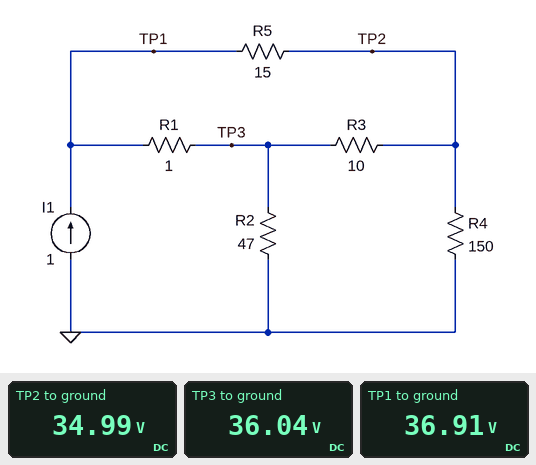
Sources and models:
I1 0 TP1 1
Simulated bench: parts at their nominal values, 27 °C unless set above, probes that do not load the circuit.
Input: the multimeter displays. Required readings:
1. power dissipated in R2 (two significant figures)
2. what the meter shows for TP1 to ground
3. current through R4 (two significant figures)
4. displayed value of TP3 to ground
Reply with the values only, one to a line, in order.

28 W
36.91 V
230 mA
36.04 V
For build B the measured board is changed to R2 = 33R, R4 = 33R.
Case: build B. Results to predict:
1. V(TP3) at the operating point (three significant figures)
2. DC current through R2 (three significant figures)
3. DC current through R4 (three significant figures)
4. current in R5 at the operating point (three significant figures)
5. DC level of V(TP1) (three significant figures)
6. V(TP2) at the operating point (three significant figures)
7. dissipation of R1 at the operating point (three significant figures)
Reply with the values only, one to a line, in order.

17.7 V
537 mA
463 mA
216 mA
18.5 V
15.3 V
614 mW
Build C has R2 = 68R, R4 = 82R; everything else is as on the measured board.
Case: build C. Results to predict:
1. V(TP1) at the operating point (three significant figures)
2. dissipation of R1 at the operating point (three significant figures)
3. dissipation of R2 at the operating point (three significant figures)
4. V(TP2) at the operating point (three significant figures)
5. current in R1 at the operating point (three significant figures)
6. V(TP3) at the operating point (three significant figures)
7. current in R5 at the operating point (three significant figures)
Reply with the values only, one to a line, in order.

39.0 V
629 mW
21.5 W
35.9 V
793 mA
38.2 V
207 mA
